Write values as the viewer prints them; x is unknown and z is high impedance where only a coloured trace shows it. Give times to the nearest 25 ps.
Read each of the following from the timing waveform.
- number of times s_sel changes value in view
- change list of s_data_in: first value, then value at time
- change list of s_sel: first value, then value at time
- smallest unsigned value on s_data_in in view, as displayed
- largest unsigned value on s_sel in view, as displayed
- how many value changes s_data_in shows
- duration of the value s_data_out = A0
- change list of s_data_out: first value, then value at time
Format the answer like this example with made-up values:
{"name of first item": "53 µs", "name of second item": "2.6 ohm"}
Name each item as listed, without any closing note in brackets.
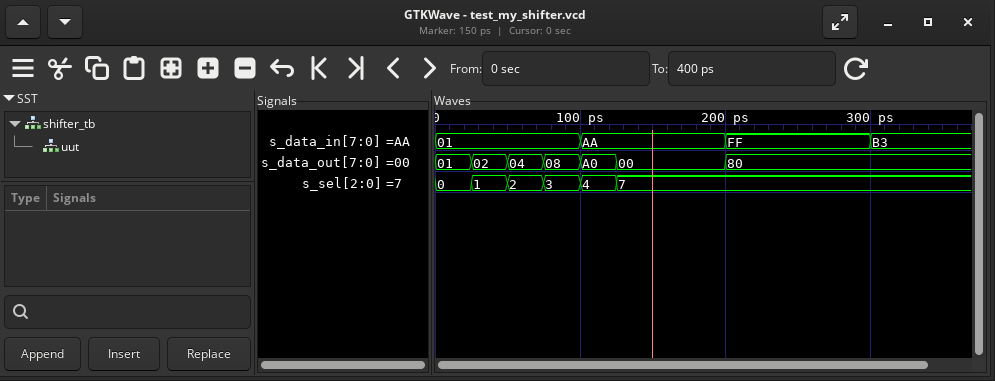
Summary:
{"number of times s_sel changes value in view": "5", "change list of s_data_in: first value, then value at time": "01, AA at 100 ps, FF at 200 ps, B3 at 300 ps", "change list of s_sel: first value, then value at time": "0, 1 at 25 ps, 2 at 50 ps, 3 at 75 ps, 4 at 100 ps, 7 at 125 ps", "smallest unsigned value on s_data_in in view, as displayed": "01", "largest unsigned value on s_sel in view, as displayed": "7", "how many value changes s_data_in shows": "3", "duration of the value s_data_out = A0": "25 ps", "change list of s_data_out: first value, then value at time": "01, 02 at 25 ps, 04 at 50 ps, 08 at 75 ps, A0 at 100 ps, 00 at 125 ps, 80 at 200 ps"}
